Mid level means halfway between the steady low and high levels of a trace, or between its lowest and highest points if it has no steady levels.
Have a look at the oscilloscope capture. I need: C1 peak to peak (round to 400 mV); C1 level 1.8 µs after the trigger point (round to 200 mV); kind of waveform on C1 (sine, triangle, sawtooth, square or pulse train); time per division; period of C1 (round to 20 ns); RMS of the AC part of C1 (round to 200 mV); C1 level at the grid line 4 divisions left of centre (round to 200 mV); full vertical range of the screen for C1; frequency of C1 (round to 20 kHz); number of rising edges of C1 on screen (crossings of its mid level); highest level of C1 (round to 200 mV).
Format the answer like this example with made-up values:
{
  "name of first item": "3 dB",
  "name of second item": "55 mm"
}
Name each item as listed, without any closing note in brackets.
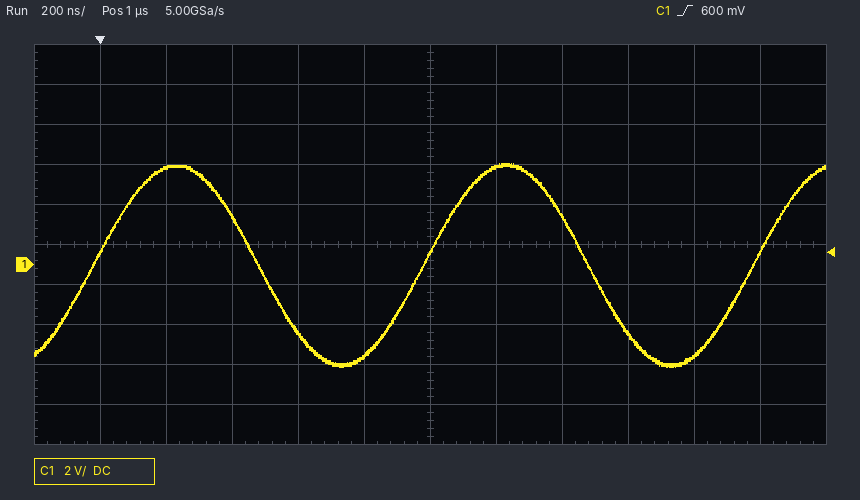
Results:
{
  "C1 peak to peak": "10.0 V",
  "C1 level 1.8 µs after the trigger point": "-4.6 V",
  "kind of waveform on C1": "sine",
  "time per division": "200 ns",
  "period of C1": "1.00 µs",
  "RMS of the AC part of C1": "3.6 V",
  "C1 level at the grid line 4 divisions left of centre": "4.8 V",
  "full vertical range of the screen for C1": "20 V",
  "frequency of C1": "1.00 MHz",
  "number of rising edges of C1 on screen": "3",
  "highest level of C1": "5.0 V"
}
